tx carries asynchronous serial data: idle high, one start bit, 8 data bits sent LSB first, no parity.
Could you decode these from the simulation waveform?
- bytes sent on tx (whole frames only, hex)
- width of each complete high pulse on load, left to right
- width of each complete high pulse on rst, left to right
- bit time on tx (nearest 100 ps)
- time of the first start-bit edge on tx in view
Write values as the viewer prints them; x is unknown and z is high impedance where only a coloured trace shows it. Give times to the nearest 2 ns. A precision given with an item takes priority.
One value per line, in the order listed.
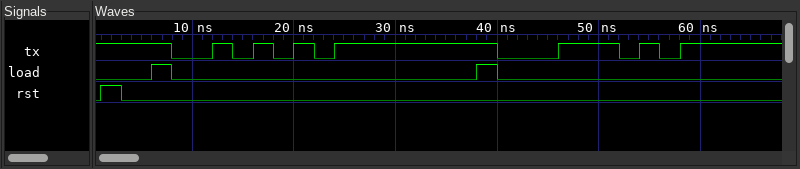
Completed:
AA, 5C
2 ns, 2 ns
2 ns
2000 ps
8 ns
